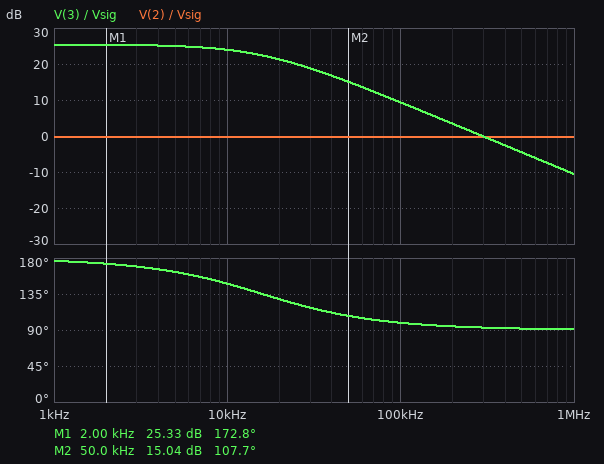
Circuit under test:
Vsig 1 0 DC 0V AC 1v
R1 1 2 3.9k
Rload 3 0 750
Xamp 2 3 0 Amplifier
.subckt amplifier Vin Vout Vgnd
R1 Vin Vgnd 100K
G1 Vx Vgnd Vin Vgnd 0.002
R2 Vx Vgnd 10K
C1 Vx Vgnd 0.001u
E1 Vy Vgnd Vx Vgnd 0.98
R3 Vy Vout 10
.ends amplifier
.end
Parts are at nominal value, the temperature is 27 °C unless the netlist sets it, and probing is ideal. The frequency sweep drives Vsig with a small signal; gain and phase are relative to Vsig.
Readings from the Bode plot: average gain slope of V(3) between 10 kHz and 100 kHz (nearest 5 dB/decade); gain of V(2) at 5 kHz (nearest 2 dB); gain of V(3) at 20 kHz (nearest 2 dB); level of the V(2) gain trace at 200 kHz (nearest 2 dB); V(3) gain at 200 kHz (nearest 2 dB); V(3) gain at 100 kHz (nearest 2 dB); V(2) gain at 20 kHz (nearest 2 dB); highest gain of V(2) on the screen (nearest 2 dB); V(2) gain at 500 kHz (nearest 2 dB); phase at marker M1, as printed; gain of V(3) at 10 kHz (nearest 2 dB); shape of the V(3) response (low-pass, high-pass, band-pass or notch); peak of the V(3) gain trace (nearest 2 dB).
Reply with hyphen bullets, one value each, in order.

- -15 dB/decade
- 0 dB
- 22 dB
- 0 dB
- 4 dB
- 10 dB
- 0 dB
- 0 dB
- 0 dB
- 172.8 deg
- 24 dB
- low-pass
- 26 dB
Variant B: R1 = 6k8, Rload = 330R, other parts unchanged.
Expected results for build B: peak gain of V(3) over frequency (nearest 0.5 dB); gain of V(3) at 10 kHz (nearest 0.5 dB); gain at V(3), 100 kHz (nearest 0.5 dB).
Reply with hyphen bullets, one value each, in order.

- 25.0 dB
- 23.5 dB
- 9.0 dB
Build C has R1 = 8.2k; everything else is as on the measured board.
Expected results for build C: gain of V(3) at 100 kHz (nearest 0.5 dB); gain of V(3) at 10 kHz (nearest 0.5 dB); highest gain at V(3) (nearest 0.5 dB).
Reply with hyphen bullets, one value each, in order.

- 9.0 dB
- 23.5 dB
- 25.0 dB
